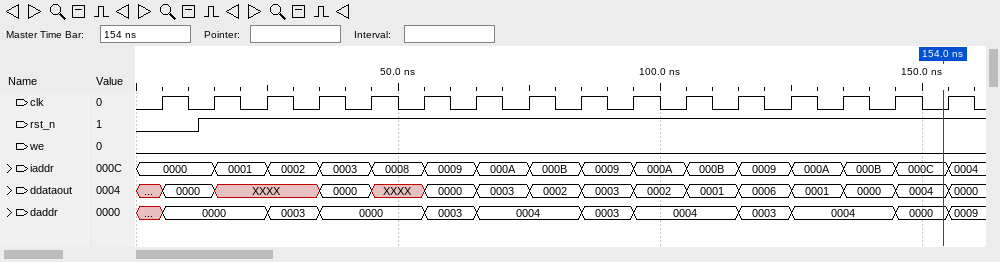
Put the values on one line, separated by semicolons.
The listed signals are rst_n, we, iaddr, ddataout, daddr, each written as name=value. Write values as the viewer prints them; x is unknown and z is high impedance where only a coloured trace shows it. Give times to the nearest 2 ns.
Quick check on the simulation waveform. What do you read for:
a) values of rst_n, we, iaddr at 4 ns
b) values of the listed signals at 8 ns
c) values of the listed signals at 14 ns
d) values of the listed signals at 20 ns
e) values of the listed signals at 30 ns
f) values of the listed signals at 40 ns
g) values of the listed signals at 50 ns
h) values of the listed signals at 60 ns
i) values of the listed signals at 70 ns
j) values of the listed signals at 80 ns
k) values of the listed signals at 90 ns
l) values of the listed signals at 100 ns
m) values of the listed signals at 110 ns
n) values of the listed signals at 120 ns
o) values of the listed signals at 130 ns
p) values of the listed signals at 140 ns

rst_n=0, we=0, iaddr=0000; rst_n=0, we=0, iaddr=0000, ddataout=0000, daddr=0000; rst_n=1, we=0, iaddr=0000, ddataout=0000, daddr=0000; rst_n=1, we=0, iaddr=0001, ddataout=XXXX, daddr=0000; rst_n=1, we=0, iaddr=0002, ddataout=XXXX, daddr=0003; rst_n=1, we=0, iaddr=0003, ddataout=0000, daddr=0000; rst_n=1, we=0, iaddr=0008, ddataout=XXXX, daddr=0000; rst_n=1, we=0, iaddr=0009, ddataout=0000, daddr=0003; rst_n=1, we=0, iaddr=000A, ddataout=0003, daddr=0004; rst_n=1, we=0, iaddr=000B, ddataout=0002, daddr=0004; rst_n=1, we=0, iaddr=0009, ddataout=0003, daddr=0003; rst_n=1, we=0, iaddr=000A, ddataout=0002, daddr=0004; rst_n=1, we=0, iaddr=000B, ddataout=0001, daddr=0004; rst_n=1, we=0, iaddr=0009, ddataout=0006, daddr=0003; rst_n=1, we=0, iaddr=000A, ddataout=0001, daddr=0004; rst_n=1, we=0, iaddr=000B, ddataout=0000, daddr=0004
